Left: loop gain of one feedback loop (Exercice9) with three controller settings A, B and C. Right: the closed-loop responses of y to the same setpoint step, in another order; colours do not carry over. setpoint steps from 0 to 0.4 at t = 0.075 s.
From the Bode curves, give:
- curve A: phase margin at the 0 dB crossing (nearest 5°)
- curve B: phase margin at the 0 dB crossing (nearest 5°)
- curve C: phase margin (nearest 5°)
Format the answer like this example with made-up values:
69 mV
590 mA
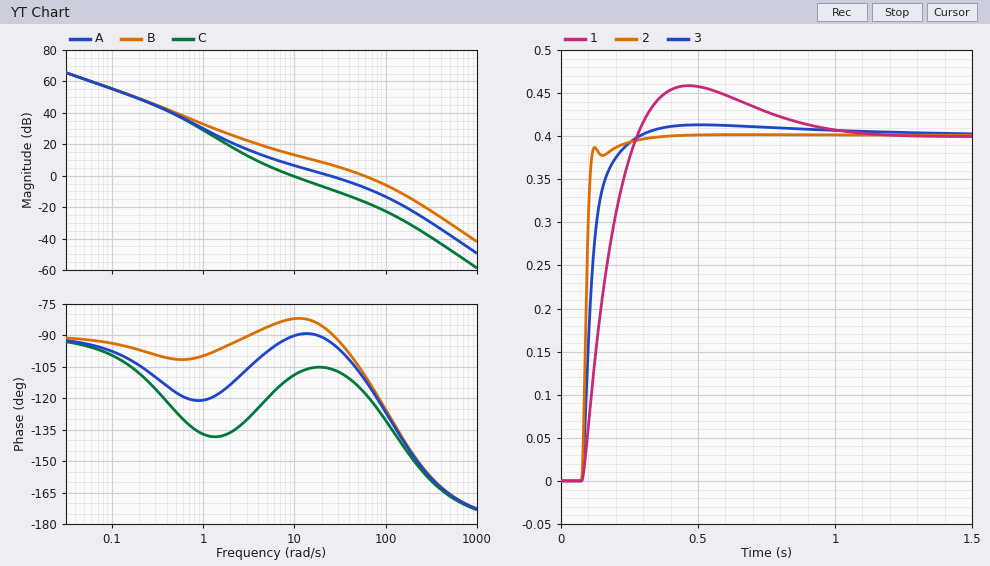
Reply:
85°
70°
70°
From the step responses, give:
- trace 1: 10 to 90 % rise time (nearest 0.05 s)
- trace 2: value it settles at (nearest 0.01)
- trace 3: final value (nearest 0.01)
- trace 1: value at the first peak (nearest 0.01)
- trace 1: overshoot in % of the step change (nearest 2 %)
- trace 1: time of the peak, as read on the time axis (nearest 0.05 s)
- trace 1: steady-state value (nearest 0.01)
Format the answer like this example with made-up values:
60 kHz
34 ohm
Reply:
0.15 s
0.40
0.40
0.46
14 %
0.45 s
0.40
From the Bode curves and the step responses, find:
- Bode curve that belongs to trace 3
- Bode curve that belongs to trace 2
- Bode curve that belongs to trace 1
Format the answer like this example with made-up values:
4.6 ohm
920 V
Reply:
A
B
C
